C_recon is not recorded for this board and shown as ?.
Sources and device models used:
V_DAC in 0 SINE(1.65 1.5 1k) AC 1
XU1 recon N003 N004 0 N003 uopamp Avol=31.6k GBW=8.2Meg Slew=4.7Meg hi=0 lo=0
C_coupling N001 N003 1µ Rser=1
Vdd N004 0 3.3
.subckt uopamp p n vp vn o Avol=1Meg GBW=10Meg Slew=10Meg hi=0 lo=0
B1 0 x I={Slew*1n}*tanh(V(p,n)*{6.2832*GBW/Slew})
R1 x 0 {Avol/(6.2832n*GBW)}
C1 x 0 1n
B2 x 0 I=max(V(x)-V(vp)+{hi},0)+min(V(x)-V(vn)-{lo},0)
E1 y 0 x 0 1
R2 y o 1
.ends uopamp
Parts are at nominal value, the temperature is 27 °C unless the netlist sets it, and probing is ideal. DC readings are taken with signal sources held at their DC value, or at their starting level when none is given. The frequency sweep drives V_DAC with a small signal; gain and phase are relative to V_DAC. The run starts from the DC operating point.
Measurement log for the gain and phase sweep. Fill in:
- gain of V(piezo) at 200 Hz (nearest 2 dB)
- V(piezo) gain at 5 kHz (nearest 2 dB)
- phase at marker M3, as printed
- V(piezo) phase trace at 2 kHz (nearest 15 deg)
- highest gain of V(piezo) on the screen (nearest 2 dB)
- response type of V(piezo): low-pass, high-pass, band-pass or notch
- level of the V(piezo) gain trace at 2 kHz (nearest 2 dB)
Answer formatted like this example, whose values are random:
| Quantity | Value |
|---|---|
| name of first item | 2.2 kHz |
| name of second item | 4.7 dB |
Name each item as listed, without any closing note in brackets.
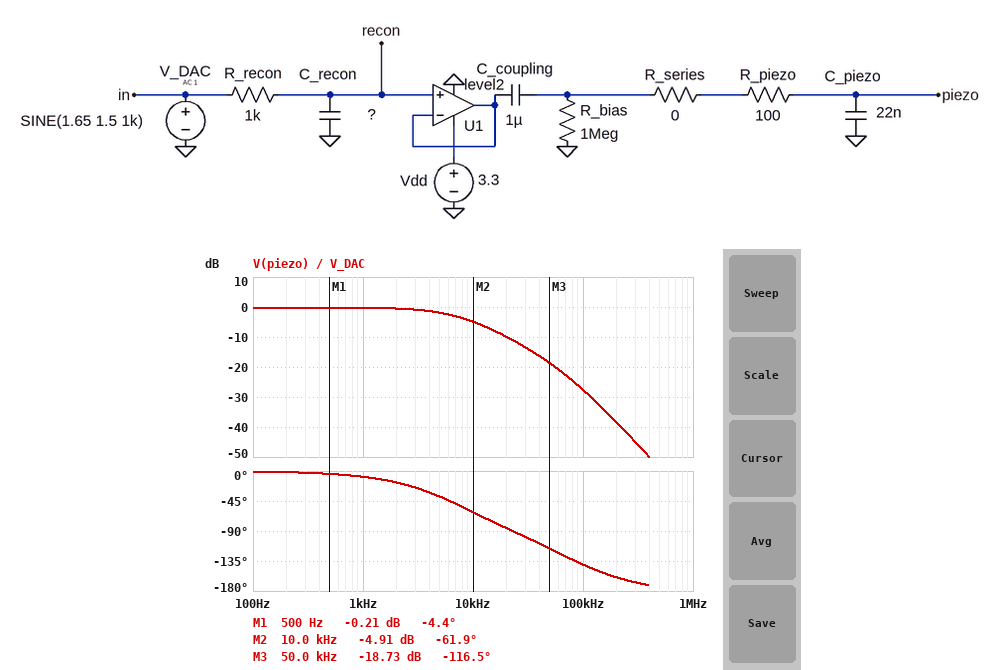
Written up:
| Quantity | Value |
|---|---|
| gain of V(piezo) at 200 Hz | 0 dB |
| V(piezo) gain at 5 kHz | -2 dB |
| phase at marker M3, as printed | -116.5 deg |
| V(piezo) phase trace at 2 kHz | -15 deg |
| highest gain of V(piezo) on the screen | 0 dB |
| response type of V(piezo): low-pass, high-pass, band-pass or notch | low-pass |
| level of the V(piezo) gain trace at 2 kHz | 0 dB |
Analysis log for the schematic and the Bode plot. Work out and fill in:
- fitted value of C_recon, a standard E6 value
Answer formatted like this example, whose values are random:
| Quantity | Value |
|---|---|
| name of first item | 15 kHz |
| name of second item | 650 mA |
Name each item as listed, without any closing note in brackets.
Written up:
| Quantity | Value |
|---|---|
| fitted value of C_recon, a standard E6 value | 22 nF |
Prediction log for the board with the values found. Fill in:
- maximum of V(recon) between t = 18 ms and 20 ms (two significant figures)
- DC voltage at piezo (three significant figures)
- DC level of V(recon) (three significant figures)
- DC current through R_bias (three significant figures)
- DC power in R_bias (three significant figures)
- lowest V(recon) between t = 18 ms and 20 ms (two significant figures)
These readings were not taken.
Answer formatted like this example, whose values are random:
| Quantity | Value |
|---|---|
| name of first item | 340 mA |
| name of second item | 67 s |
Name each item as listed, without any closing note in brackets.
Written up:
| Quantity | Value |
|---|---|
| maximum of V(recon) between t = 18 ms and 20 ms | 3.1 V |
| DC voltage at piezo | 1.59 V |
| DC level of V(recon) | 1.65 V |
| DC current through R_bias | 1.61 µA |
| DC power in R_bias | 2.60 µW |
| lowest V(recon) between t = 18 ms and 20 ms | 160 mV |
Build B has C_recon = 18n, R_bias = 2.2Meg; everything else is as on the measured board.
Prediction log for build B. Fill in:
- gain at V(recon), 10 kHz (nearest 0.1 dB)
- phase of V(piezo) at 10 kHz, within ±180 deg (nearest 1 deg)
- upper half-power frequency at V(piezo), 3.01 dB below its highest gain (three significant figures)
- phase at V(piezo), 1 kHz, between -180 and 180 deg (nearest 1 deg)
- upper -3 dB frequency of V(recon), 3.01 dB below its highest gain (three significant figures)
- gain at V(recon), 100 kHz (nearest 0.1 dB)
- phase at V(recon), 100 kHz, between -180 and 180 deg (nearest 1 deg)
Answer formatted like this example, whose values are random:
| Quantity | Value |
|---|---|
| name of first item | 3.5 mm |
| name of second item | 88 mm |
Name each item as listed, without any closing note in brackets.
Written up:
| Quantity | Value |
|---|---|
| gain at V(recon), 10 kHz | -3.6 dB |
| phase of V(piezo) at 10 kHz, within ±180 deg | -56 deg |
| upper half-power frequency at V(piezo), 3.01 dB below its highest gain | 8.72 kHz |
| phase at V(piezo), 1 kHz, between -180 and 180 deg | -7 deg |
| upper -3 dB frequency of V(recon), 3.01 dB below its highest gain | 8.84 kHz |
| gain at V(recon), 100 kHz | -21.1 dB |
| phase at V(recon), 100 kHz, between -180 and 180 deg | -85 deg |
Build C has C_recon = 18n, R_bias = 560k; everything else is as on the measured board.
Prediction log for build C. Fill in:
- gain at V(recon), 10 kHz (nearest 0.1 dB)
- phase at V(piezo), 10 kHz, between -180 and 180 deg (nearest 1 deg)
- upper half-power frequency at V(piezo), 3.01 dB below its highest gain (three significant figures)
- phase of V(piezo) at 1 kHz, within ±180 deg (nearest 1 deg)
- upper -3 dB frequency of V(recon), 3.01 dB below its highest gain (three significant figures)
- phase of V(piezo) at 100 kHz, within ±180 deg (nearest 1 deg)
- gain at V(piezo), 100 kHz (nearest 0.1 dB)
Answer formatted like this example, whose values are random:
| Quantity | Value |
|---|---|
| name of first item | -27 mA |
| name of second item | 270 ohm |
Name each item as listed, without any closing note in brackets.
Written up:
| Quantity | Value |
|---|---|
| gain at V(recon), 10 kHz | -3.6 dB |
| phase at V(piezo), 10 kHz, between -180 and 180 deg | -56 deg |
| upper half-power frequency at V(piezo), 3.01 dB below its highest gain | 8.72 kHz |
| phase of V(piezo) at 1 kHz, within ±180 deg | -7 deg |
| upper -3 dB frequency of V(recon), 3.01 dB below its highest gain | 8.84 kHz |
| phase of V(piezo) at 100 kHz, within ±180 deg | -139 deg |
| gain at V(piezo), 100 kHz | -25.9 dB |
